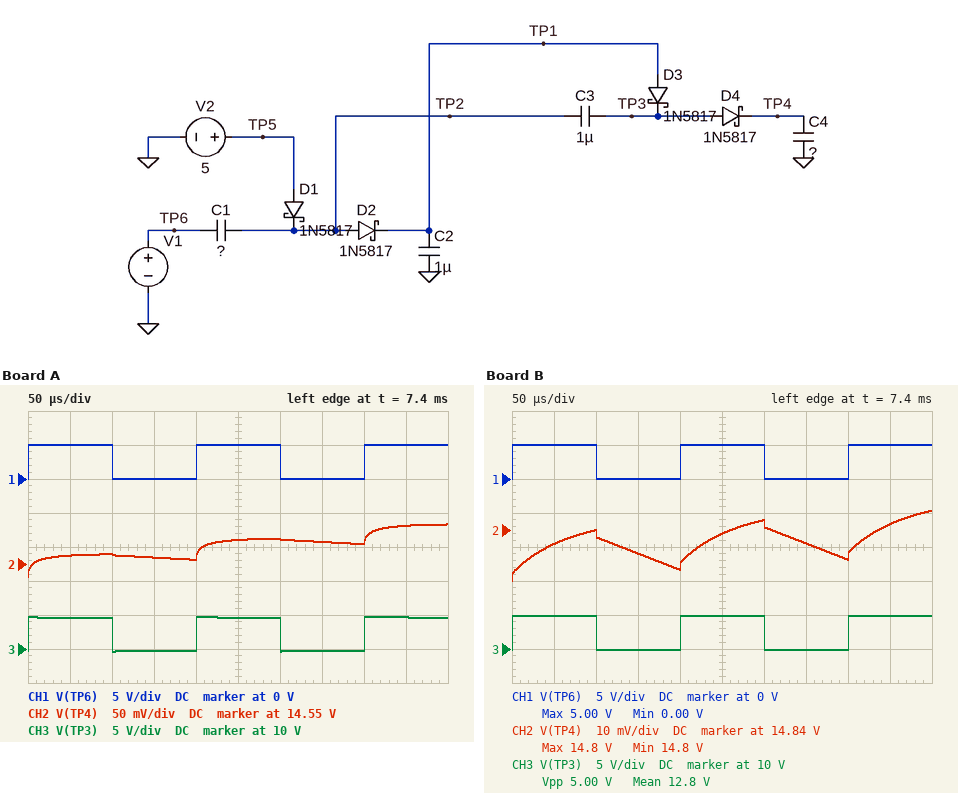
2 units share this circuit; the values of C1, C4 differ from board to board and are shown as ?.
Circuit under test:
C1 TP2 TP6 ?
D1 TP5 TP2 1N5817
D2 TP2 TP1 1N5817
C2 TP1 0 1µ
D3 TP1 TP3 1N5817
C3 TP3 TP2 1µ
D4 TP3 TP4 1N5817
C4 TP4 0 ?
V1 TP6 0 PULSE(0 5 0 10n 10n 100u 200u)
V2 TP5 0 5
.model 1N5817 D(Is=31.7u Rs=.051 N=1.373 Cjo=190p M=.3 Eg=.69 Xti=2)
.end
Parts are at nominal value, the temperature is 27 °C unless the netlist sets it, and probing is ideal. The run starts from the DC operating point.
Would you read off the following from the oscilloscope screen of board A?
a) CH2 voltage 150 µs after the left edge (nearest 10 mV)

14.56 V
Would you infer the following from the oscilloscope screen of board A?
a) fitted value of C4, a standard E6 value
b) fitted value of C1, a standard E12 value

470 nF
470 nF
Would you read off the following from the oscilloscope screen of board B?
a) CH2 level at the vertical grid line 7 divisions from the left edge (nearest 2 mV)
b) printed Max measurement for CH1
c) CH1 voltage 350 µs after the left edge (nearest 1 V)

14.836 V
5.00 V
0 V
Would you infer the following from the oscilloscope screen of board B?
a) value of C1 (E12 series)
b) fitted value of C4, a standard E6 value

1.8 µF
330 nF
